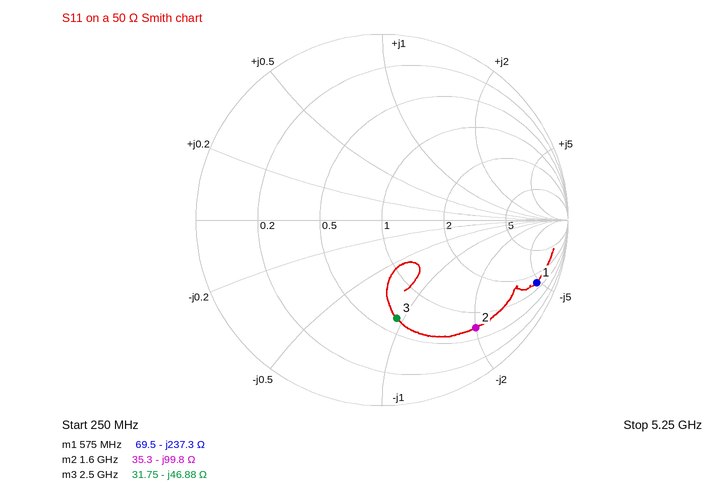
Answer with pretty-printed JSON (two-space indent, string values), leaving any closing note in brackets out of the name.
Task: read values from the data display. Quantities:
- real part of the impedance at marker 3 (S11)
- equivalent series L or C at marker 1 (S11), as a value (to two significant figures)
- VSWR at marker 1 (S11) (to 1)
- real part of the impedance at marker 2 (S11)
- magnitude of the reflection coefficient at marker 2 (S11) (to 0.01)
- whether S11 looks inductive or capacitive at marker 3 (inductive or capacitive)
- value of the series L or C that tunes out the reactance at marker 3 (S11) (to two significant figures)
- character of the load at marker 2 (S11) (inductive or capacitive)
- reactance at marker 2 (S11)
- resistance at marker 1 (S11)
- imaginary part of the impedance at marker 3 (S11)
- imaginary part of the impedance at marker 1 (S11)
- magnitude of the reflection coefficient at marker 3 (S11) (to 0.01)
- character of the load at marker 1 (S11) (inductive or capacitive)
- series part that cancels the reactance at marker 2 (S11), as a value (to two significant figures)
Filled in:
{
  "real part of the impedance at marker 3": "31.75 Ω",
  "equivalent series L or C at marker 1 (S11), as a value": "1.2 pF",
  "VSWR at marker 1 (S11)": "18",
  "real part of the impedance at marker 2": "35.3 Ω",
  "magnitude of the reflection coefficient at marker 2 (S11)": "0.77",
  "whether S11 looks inductive or capacitive at marker 3": "capacitive",
  "value of the series L or C that tunes out the reactance at marker 3 (S11)": "3.0 nH",
  "character of the load at marker 2 (S11)": "capacitive",
  "reactance at marker 2": "-99.8 Ω",
  "resistance at marker 1": "69.5 Ω",
  "imaginary part of the impedance at marker 3": "-46.88 Ω",
  "imaginary part of the impedance at marker 1": "-237.3 Ω",
  "magnitude of the reflection coefficient at marker 3 (S11)": "0.53",
  "character of the load at marker 1 (S11)": "capacitive",
  "series part that cancels the reactance at marker 2 (S11), as a value": "9.9 nH"
}
